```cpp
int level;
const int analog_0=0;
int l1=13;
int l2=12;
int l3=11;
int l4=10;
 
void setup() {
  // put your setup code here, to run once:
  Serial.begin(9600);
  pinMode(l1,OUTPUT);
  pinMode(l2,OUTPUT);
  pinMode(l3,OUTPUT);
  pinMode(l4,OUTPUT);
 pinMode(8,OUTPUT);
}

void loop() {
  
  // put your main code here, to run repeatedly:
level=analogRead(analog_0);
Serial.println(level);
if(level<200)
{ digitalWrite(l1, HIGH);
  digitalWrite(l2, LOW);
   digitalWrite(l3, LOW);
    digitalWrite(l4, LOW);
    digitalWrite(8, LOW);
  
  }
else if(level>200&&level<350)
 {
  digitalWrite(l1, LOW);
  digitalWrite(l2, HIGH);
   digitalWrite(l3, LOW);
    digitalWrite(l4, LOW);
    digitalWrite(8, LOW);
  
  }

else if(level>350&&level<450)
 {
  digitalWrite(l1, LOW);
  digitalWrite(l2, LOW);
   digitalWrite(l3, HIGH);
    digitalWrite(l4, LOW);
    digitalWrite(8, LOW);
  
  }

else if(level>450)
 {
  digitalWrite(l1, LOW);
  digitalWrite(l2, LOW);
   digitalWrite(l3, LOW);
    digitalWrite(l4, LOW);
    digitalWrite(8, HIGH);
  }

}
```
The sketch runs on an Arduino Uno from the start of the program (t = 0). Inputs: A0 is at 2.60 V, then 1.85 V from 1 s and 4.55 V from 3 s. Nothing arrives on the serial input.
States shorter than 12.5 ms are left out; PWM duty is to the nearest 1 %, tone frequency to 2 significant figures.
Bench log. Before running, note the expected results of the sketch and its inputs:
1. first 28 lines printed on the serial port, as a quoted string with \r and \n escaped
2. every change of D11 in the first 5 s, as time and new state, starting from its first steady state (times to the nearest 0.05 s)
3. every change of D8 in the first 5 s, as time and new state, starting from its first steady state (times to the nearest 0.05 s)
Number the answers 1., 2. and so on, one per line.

1. "532\r\n532\r\n532\r\n532\r\n532\r\n532\r\n532\r\n532\r\n532\r\n532\r\n532\r\n532\r\n532\r\n532\r\n532\r\n532\r\n532\r\n532\r\n532\r\n532\r\n532\r\n532\r\n532\r\n532\r\n532\r\n532\r\n532\r\n532\r\n"
2. 0 s low; 1 s high; 3 s low
3. 0 s high; 1 s low; 3 s high
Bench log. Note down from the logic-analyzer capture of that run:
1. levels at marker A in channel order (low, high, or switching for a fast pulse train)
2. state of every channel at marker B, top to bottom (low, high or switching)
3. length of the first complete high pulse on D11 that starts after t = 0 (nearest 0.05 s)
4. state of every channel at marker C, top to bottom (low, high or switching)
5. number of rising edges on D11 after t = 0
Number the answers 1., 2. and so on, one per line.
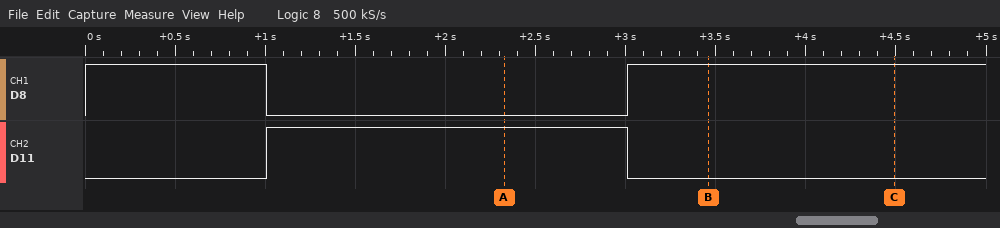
1. D8 low, D11 high
2. D8 high, D11 low
3. 2.00 s
4. D8 high, D11 low
5. 1
